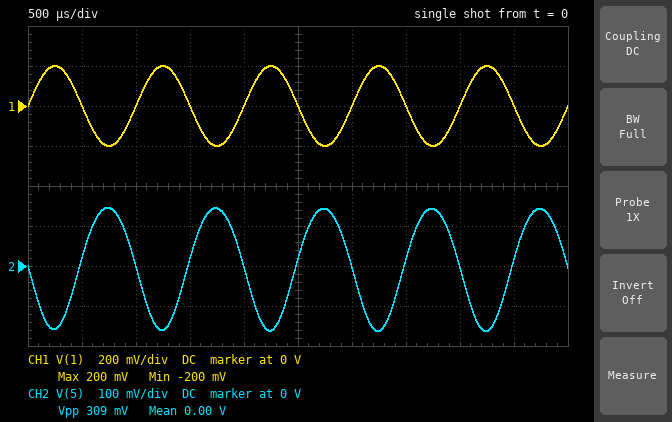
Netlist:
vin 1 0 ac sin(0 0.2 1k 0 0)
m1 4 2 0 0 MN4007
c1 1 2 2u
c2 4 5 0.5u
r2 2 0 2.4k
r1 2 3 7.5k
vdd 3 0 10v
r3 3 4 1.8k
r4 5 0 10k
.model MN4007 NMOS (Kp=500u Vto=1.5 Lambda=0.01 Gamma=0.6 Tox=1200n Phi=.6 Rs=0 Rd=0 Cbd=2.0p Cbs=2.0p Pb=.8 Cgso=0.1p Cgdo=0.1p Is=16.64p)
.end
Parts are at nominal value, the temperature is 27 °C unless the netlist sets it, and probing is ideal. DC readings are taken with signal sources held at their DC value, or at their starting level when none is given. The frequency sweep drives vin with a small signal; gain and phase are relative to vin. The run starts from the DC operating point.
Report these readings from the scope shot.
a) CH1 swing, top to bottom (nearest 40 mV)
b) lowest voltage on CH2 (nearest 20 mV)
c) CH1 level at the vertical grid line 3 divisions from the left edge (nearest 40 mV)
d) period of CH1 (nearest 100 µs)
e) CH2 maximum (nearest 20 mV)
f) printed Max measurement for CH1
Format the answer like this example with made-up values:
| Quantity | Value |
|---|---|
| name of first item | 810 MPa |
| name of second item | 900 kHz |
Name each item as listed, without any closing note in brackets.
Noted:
| Quantity | Value |
|---|---|
| CH1 swing, top to bottom | 400 mV |
| lowest voltage on CH2 | -160 mV |
| CH1 level at the vertical grid line 3 divisions from the left edge | 0 V |
| period of CH1 | 1.0 ms |
| CH2 maximum | 140 mV |
| printed Max measurement for CH1 | 200 mV |
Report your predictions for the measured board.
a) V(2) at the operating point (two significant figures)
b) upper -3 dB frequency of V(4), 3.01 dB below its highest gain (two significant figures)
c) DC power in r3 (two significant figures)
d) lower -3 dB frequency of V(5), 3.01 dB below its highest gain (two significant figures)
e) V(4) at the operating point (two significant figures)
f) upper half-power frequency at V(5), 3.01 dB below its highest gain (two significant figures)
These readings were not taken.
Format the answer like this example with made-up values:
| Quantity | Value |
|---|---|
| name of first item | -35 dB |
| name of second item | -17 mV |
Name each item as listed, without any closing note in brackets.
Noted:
| Quantity | Value |
|---|---|
| V(2) at the operating point | 2.4 V |
| upper -3 dB frequency of V(4), 3.01 dB below its highest gain | 190 MHz |
| DC power in r3 | 99 µW |
| lower -3 dB frequency of V(5), 3.01 dB below its highest gain | 56 Hz |
| V(4) at the operating point | 9.6 V |
| upper half-power frequency at V(5), 3.01 dB below its highest gain | 190 MHz |
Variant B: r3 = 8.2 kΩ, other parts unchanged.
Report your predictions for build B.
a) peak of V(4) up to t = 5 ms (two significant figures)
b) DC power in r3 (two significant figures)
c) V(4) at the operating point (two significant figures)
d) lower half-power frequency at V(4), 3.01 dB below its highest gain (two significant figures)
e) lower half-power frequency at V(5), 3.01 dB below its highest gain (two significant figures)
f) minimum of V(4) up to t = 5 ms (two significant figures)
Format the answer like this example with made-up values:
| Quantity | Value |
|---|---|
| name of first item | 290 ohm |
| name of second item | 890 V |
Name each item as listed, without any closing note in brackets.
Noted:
| Quantity | Value |
|---|---|
| peak of V(4) up to t = 5 ms | 8.5 V |
| DC power in r3 | 440 µW |
| V(4) at the operating point | 8.1 V |
| lower half-power frequency at V(4), 3.01 dB below its highest gain | 30 Hz |
| lower half-power frequency at V(5), 3.01 dB below its highest gain | 50 Hz |
| minimum of V(4) up to t = 5 ms | 7.6 V |
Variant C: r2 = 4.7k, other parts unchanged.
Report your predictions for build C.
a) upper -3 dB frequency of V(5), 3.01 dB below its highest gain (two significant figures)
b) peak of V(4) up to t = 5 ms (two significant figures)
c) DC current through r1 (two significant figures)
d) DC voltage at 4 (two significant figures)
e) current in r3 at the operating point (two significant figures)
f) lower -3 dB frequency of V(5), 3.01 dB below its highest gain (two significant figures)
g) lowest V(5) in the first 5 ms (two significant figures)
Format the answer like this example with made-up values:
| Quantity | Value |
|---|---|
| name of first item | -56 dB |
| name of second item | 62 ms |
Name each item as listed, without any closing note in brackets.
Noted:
| Quantity | Value |
|---|---|
| upper -3 dB frequency of V(5), 3.01 dB below its highest gain | 170 MHz |
| peak of V(4) up to t = 5 ms | 7.7 V |
| DC current through r1 | 820 µA |
| DC voltage at 4 | 7.3 V |
| current in r3 at the operating point | 1.5 mA |
| lower -3 dB frequency of V(5), 3.01 dB below its highest gain | 42 Hz |
| lowest V(5) in the first 5 ms | -380 mV |
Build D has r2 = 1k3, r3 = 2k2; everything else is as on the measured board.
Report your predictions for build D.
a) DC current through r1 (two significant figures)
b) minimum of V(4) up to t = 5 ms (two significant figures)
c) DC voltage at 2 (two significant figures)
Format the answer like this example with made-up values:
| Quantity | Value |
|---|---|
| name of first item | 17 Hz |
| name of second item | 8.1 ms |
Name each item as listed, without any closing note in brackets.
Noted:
| Quantity | Value |
|---|---|
| DC current through r1 | 1.1 mA |
| minimum of V(4) up to t = 5 ms | 10 V |
| DC voltage at 2 | 1.5 V |
